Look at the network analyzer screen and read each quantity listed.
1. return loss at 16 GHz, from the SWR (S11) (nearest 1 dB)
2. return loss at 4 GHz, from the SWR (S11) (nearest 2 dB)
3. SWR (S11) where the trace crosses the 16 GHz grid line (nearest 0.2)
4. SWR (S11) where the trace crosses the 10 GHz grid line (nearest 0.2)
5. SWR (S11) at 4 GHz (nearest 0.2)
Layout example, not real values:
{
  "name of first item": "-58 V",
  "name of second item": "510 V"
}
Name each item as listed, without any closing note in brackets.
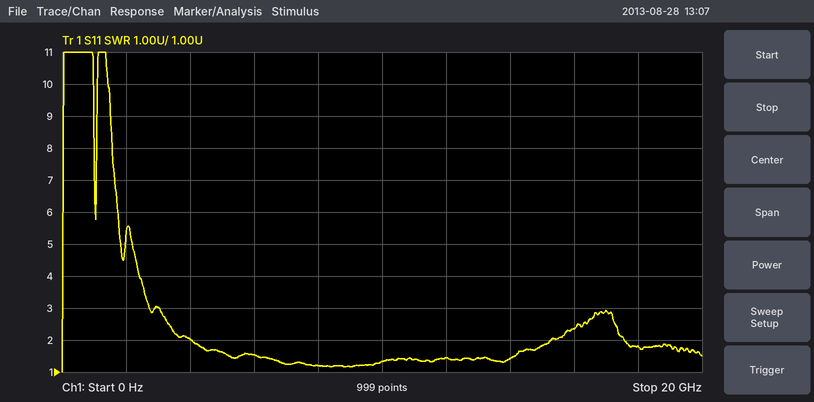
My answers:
{
  "return loss at 16 GHz, from the SWR (S11)": "8 dB",
  "return loss at 4 GHz, from the SWR (S11)": "10 dB",
  "SWR (S11) where the trace crosses the 16 GHz grid line": "2.4",
  "SWR (S11) where the trace crosses the 10 GHz grid line": "1.4",
  "SWR (S11) at 4 GHz": "2.0"
}
